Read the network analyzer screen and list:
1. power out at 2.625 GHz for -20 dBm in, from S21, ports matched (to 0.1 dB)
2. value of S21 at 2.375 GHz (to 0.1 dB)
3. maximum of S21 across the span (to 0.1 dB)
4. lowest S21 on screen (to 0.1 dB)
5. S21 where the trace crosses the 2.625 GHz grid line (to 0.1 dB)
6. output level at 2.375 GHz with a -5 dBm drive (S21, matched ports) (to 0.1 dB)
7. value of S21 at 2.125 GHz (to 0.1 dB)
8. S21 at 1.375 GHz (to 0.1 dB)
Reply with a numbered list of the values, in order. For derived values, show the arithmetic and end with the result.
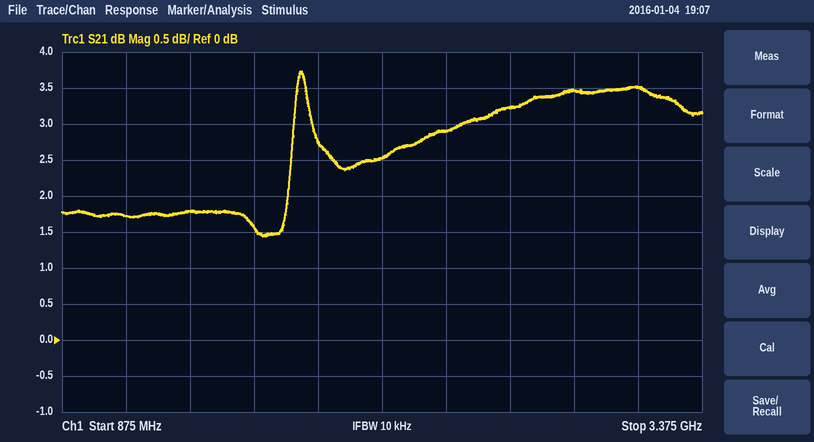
1. -20 dBm + (3.2 dB) = -16.8 dBm
2. 2.9 dB
3. 3.7 dB
4. 1.4 dB
5. 3.2 dB
6. -5 dBm + (2.9 dB) = -2.1 dBm
7. 2.5 dB
8. 1.8 dB
